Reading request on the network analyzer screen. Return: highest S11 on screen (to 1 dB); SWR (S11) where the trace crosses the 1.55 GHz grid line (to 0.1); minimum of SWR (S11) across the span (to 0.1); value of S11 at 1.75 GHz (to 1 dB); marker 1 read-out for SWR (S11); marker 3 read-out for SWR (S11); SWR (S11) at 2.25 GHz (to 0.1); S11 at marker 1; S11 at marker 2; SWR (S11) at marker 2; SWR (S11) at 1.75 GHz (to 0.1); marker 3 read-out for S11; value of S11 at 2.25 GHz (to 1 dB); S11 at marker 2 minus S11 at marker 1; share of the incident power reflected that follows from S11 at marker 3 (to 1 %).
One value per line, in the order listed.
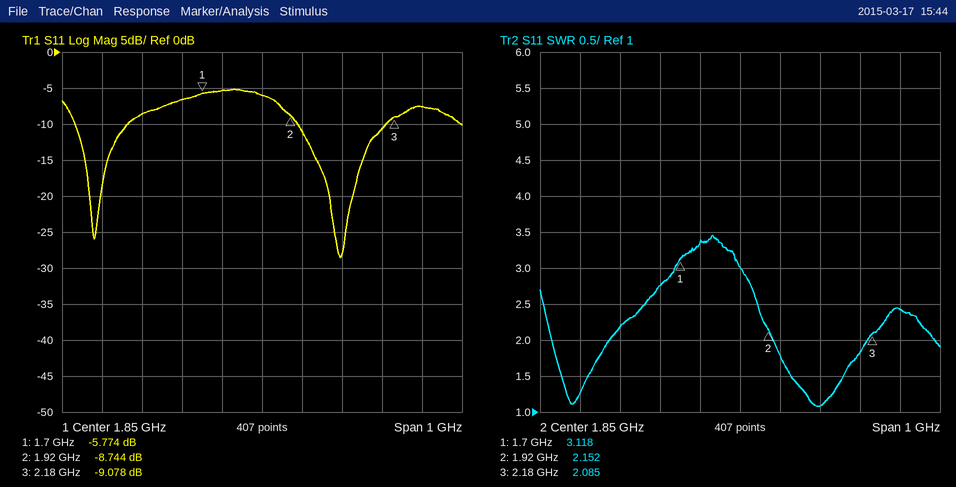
-5 dB
2.2
1.1
-5 dB
3.118
2.085
2.4
-5.774 dB
-8.744 dB
2.152
3.4
-9.078 dB
-8 dB
-2.970 dB
12 %
